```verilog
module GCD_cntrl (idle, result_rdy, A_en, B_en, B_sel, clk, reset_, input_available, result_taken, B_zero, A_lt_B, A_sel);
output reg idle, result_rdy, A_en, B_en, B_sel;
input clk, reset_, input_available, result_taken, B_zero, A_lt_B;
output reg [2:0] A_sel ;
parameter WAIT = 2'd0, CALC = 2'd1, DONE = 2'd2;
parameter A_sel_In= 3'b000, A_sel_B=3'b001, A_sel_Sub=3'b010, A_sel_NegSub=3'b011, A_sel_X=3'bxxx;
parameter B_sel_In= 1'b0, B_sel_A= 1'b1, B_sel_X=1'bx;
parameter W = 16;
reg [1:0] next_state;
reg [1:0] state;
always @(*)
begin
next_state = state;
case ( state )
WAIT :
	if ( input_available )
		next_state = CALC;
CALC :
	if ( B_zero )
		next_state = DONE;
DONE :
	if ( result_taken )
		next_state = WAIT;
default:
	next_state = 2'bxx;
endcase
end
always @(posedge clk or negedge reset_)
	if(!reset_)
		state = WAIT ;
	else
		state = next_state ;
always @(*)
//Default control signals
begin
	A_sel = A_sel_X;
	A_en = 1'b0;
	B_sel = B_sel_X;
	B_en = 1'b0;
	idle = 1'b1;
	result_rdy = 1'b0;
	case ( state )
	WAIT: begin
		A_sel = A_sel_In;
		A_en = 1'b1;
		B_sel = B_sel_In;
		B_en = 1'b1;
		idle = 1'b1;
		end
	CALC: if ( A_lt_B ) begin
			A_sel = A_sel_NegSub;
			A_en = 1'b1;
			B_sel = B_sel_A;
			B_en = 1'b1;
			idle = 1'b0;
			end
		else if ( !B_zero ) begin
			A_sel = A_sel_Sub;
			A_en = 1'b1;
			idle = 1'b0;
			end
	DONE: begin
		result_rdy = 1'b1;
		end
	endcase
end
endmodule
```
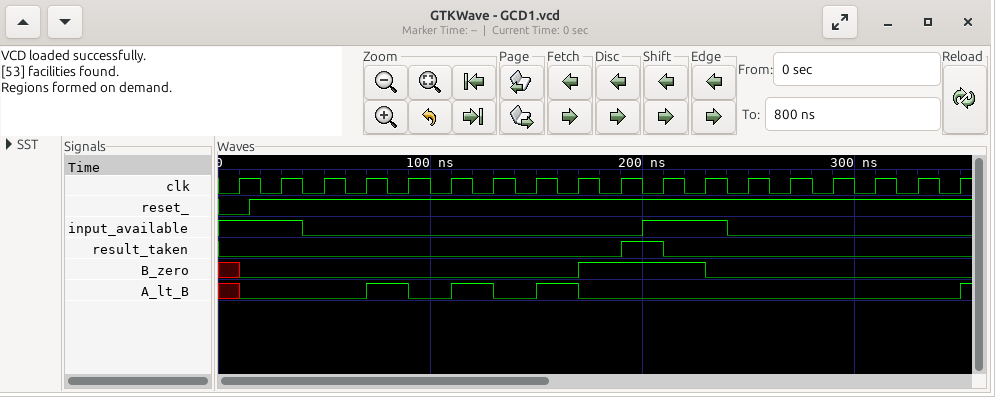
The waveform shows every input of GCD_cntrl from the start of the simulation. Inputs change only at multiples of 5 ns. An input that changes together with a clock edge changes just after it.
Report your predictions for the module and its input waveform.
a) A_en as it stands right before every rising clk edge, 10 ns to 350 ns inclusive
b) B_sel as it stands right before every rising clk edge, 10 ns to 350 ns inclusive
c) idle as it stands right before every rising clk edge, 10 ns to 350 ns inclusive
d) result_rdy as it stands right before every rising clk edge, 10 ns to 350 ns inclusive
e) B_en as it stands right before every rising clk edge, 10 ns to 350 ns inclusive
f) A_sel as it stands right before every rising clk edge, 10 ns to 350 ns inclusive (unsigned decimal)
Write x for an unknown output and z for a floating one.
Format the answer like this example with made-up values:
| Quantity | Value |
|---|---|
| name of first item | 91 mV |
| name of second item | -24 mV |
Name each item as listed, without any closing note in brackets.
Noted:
| Quantity | Value |
|---|---|
| A_en as it stands right before every rising clk edge, 10 ns to 350 ns inclusive | 1 1 1 1 1 1 1 1 1 0 0 1 1 1 1 1 1 1 |
| B_sel as it stands right before every rising clk edge, 10 ns to 350 ns inclusive | 0 0 x x 1 x 1 x 1 x x 0 x x x x x x |
| idle as it stands right before every rising clk edge, 10 ns to 350 ns inclusive | 1 1 0 0 0 0 0 0 0 1 1 1 0 0 0 0 0 0 |
| result_rdy as it stands right before every rising clk edge, 10 ns to 350 ns inclusive | 0 0 0 0 0 0 0 0 0 0 1 0 0 0 0 0 0 0 |
| B_en as it stands right before every rising clk edge, 10 ns to 350 ns inclusive | 1 1 0 0 1 0 1 0 1 0 0 1 0 0 0 0 0 0 |
| A_sel as it stands right before every rising clk edge, 10 ns to 350 ns inclusive | 0, 0, 2, 2, 3, 2, 3, 2, 3, x, x, 0, 2, 2, 2, 2, 2, 2 |
